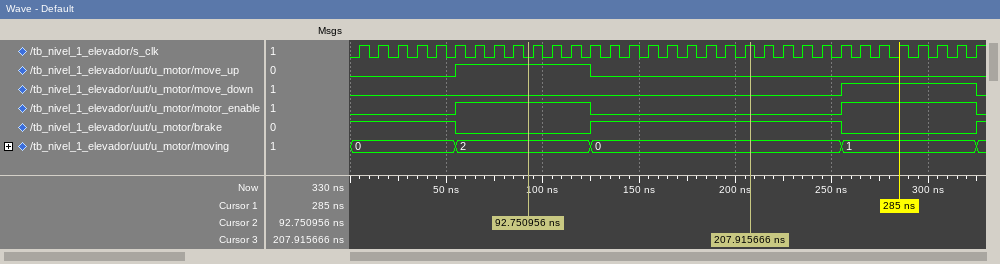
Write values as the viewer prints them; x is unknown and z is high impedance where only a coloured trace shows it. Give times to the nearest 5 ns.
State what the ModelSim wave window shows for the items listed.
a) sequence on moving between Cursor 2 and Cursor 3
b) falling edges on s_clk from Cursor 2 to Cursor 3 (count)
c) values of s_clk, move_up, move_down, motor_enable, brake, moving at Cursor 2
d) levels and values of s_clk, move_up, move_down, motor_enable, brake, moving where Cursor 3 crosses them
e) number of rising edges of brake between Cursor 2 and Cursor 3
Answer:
2, 0
11
s_clk=0, move_up=1, move_down=0, motor_enable=1, brake=0, moving=2
s_clk=1, move_up=0, move_down=0, motor_enable=0, brake=1, moving=0
1
